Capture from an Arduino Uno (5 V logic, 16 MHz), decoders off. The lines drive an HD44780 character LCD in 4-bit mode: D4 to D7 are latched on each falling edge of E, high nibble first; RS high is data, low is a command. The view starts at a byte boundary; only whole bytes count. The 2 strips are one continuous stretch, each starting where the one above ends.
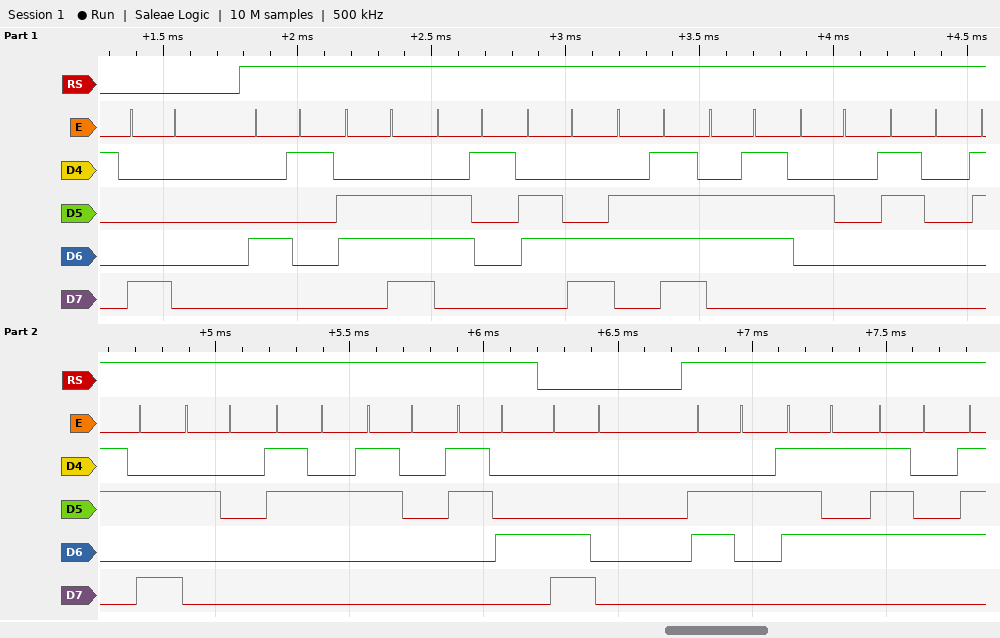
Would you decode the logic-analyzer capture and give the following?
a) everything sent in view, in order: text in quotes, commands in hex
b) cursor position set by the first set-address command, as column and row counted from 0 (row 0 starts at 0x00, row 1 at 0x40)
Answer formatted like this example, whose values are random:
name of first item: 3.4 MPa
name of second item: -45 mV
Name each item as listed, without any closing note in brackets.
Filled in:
everything sent in view, in order: text in quotes, commands in hex: 0x80 "Analog 0: 204" 0xC0 "but"
cursor position set by the first set-address command, as column and row counted from 0: column 0, row 0
